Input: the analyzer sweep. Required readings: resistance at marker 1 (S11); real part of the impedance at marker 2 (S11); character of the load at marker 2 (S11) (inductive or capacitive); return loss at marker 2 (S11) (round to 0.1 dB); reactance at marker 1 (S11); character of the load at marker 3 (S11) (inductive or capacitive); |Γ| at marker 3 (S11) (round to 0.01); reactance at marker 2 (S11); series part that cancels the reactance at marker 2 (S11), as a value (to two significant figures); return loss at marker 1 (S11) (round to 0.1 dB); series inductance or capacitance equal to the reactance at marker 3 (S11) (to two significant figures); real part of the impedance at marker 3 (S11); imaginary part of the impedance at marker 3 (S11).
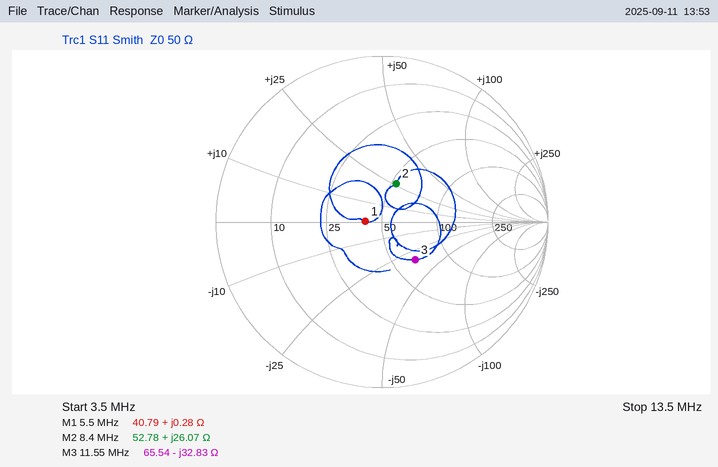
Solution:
40.79 Ω
52.78 Ω
inductive
12.1 dB
+0.28 Ω
capacitive
0.30
+26.07 Ω
730 pF
19.9 dB
420 pF
65.54 Ω
-32.83 Ω
